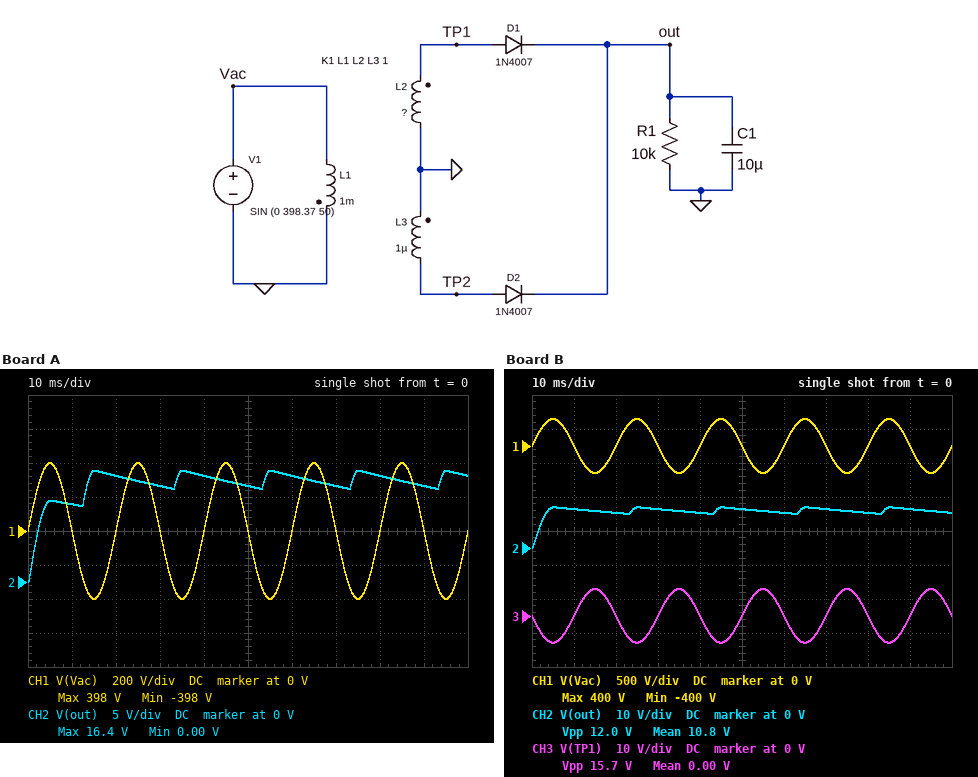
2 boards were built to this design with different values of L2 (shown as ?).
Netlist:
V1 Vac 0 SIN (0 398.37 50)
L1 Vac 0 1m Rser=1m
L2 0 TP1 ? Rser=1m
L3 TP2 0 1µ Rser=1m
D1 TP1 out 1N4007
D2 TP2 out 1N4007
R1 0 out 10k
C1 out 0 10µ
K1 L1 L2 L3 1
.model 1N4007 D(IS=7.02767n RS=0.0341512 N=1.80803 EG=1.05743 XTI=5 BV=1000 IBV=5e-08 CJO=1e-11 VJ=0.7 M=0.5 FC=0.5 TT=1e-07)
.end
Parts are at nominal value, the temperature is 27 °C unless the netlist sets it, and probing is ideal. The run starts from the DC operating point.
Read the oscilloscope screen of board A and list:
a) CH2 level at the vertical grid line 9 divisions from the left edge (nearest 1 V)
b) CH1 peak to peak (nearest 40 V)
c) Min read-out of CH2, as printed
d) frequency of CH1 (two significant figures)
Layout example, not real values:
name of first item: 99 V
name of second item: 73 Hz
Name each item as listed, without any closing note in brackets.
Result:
CH2 level at the vertical grid line 9 divisions from the left edge: 14 V
CH1 peak to peak: 800 V
Min read-out of CH2, as printed: 0.00 V
frequency of CH1: 50 Hz
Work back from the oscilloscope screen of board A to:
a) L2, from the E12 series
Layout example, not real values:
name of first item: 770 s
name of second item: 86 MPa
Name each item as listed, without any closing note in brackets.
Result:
L2, from the E12 series: 1.8 µH
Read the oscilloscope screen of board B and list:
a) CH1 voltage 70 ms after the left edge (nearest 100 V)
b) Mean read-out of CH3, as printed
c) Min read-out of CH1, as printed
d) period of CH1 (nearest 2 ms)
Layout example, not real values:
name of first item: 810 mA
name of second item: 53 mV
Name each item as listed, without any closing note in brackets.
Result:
CH1 voltage 70 ms after the left edge: 0 V
Mean read-out of CH3, as printed: 0.00 V
Min read-out of CH1, as printed: -400 V
period of CH1: 20 ms
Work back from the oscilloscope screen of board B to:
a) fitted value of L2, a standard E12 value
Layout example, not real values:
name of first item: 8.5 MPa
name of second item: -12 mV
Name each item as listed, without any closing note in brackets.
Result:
fitted value of L2, a standard E12 value: 390 nH
